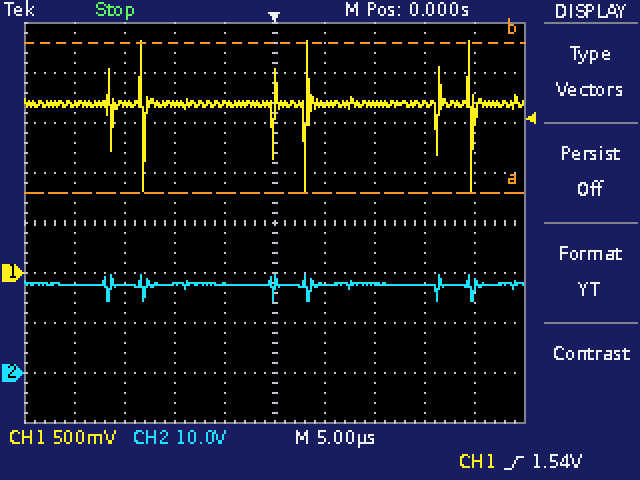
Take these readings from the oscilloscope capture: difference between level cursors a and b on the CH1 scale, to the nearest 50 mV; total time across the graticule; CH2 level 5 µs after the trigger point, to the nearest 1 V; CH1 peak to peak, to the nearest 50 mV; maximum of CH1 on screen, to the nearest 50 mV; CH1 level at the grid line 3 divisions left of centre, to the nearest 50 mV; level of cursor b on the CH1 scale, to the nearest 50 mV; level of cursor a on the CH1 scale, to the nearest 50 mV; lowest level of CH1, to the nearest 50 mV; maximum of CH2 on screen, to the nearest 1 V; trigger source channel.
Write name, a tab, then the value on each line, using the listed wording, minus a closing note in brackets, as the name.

difference between level cursors a and b on the CH1 scale, to the nearest 50 mV	1.50 V
total time across the graticule	50 µs
CH2 level 5 µs after the trigger point, to the nearest 1 V	18 V
CH1 peak to peak, to the nearest 50 mV	1.50 V
maximum of CH1 on screen, to the nearest 50 mV	2.30 V
CH1 level at the grid line 3 divisions left of centre, to the nearest 50 mV	1.70 V
level of cursor b on the CH1 scale, to the nearest 50 mV	2.30 V
level of cursor a on the CH1 scale, to the nearest 50 mV	800 mV
lowest level of CH1, to the nearest 50 mV	800 mV
maximum of CH2 on screen, to the nearest 1 V	20 V
trigger source channel	CH1
